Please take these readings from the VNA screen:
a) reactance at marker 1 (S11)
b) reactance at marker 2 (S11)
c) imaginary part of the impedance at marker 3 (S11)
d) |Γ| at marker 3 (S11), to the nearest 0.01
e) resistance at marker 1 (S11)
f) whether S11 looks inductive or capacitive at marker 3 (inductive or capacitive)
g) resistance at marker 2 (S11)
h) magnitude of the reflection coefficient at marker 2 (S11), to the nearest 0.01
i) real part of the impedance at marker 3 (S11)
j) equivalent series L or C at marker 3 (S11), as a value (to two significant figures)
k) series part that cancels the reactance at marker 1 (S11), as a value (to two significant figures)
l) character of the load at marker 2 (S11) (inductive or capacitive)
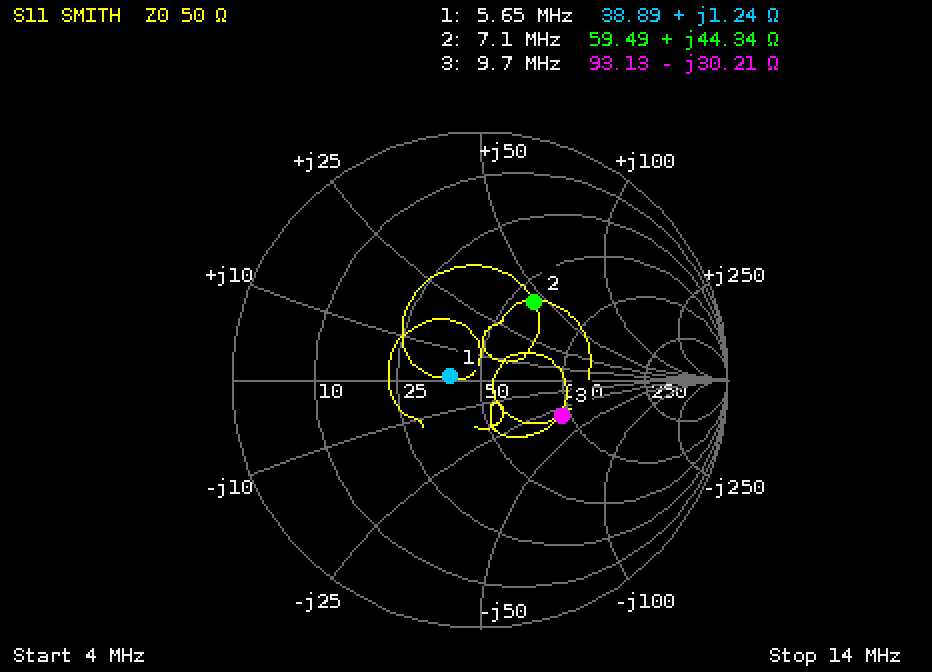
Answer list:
+1.24 Ω
+44.34 Ω
-30.21 Ω
0.36
38.89 Ω
capacitive
59.49 Ω
0.38
93.13 Ω
540 pF
23 nF
inductive
